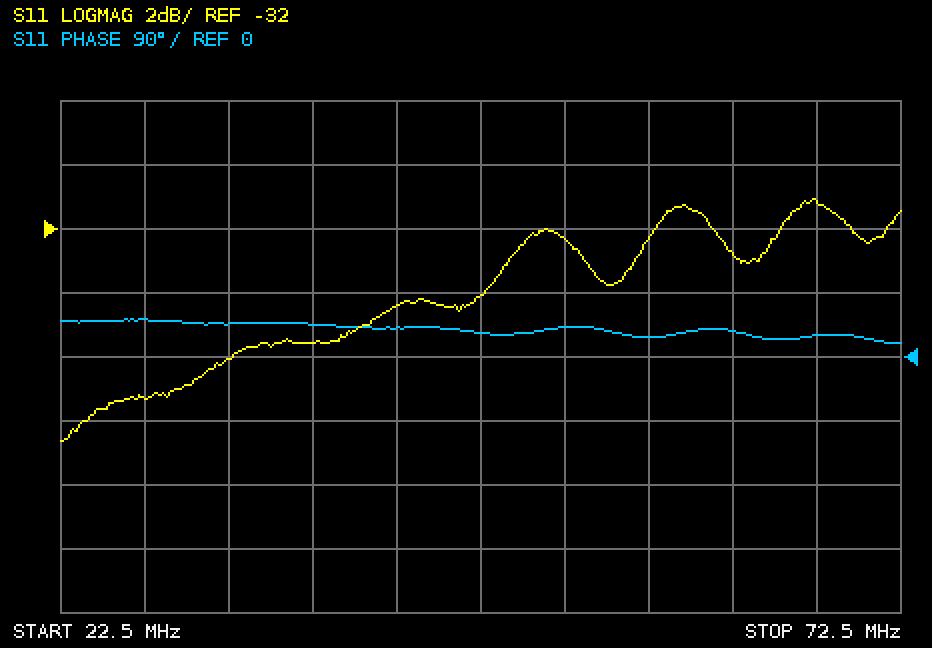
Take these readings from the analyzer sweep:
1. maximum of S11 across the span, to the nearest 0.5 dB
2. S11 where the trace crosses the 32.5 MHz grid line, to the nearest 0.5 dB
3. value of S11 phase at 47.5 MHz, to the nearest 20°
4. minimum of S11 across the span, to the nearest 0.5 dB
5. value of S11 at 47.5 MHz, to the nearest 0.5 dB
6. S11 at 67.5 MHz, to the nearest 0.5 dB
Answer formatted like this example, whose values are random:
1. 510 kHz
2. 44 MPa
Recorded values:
1. -31.0 dB
2. -36.0 dB
3. 40°
4. -38.5 dB
5. -34.0 dB
6. -31.0 dB
